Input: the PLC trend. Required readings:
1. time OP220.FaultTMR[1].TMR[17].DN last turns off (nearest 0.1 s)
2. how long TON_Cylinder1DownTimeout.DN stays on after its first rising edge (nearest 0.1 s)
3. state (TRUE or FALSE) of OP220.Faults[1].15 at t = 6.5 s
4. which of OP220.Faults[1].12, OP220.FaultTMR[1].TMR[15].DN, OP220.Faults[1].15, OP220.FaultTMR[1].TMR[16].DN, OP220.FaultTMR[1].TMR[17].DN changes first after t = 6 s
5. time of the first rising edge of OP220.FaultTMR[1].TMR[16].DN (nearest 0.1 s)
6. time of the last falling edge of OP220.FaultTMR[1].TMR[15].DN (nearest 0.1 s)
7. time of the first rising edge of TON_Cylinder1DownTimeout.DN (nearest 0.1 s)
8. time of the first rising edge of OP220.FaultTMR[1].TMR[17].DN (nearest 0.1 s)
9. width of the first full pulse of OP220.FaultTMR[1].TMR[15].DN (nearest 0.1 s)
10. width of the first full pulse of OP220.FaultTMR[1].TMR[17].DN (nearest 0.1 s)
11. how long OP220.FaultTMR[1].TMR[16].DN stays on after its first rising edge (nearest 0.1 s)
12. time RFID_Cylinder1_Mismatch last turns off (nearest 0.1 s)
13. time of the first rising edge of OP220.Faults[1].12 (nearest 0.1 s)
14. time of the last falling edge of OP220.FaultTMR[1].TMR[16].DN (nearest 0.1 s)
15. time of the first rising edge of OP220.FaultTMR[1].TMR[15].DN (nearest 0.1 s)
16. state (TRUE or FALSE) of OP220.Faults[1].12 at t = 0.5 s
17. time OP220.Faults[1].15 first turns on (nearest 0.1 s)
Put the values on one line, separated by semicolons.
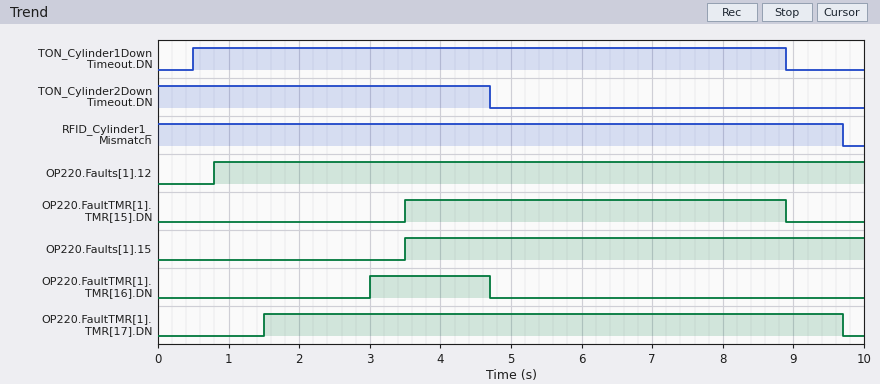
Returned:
9.7 s; 8.4 s; TRUE; OP220.FaultTMR[1].TMR[15].DN; 3.0 s; 8.9 s; 0.5 s; 1.5 s; 5.4 s; 8.2 s; 1.7 s; 9.7 s; 0.8 s; 4.7 s; 3.5 s; FALSE; 3.5 s
